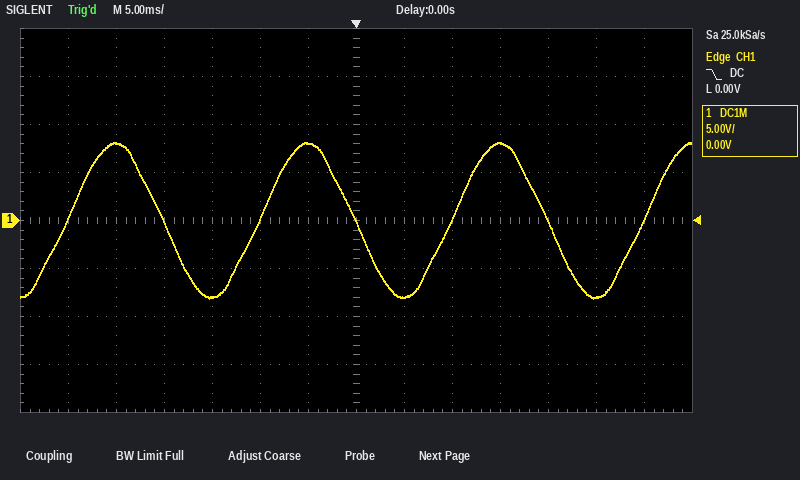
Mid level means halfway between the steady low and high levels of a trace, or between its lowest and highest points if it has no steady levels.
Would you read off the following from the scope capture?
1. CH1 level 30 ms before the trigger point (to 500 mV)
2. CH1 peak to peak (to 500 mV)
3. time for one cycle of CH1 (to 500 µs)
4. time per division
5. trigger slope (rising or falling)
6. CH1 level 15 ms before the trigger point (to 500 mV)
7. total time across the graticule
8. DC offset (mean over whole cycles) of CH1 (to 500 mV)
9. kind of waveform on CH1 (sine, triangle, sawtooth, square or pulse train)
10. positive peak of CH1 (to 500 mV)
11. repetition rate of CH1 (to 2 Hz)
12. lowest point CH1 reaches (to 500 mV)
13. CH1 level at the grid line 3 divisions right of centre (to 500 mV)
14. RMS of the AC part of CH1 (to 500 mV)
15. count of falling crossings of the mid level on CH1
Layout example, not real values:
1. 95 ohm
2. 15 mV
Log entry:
1. 0.0 V
2. 16.0 V
3. 20.0 ms
4. 5 ms
5. falling
6. -8.0 V
7. 70 ms
8. 0.0 V
9. sine
10. 8.0 V
11. 50 Hz
12. -8.0 V
13. 8.0 V
14. 5.5 V
15. 3
